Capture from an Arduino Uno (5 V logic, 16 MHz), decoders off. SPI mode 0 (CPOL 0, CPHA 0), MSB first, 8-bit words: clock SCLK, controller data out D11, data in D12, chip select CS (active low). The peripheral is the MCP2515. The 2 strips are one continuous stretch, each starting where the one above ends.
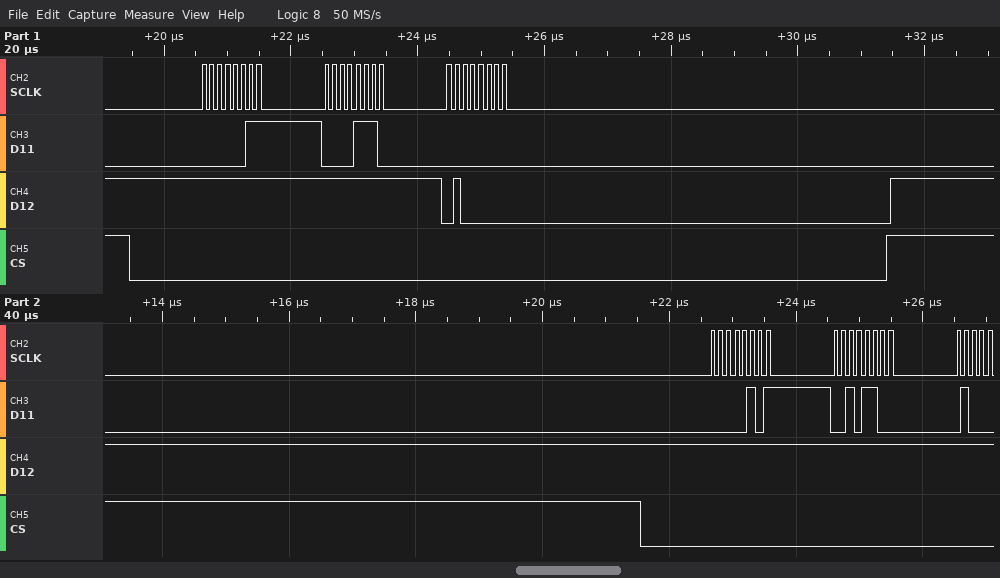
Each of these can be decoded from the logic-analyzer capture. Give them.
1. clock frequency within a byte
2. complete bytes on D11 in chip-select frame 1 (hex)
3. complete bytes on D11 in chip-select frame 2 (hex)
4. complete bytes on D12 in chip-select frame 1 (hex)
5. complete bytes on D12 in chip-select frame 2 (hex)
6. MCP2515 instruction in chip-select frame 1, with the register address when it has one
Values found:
8 MHz
0x03 0x0E 0x00
0x05 0x2C
0xFF 0xFF 0x40
0xFF 0xFF
READ 0x0E
